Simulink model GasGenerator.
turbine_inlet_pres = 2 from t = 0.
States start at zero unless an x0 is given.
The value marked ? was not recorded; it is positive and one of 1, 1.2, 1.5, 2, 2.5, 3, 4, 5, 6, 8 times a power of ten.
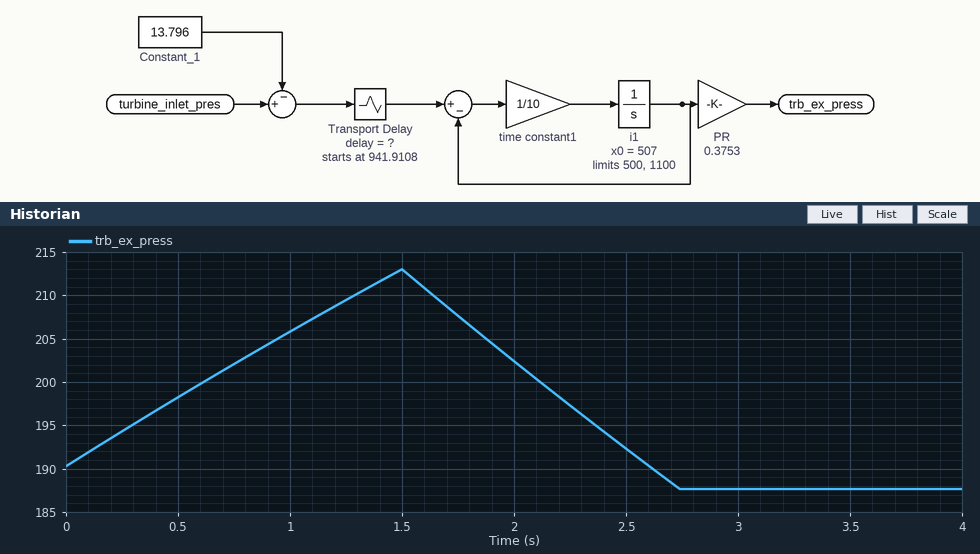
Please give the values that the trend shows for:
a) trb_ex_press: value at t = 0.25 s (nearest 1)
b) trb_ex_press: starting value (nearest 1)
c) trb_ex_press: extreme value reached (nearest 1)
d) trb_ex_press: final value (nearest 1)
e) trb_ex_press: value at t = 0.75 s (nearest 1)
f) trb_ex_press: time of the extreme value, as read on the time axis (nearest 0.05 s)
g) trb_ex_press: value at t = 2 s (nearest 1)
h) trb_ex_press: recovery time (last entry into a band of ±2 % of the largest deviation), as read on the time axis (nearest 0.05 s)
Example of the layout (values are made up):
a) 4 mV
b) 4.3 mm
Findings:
a) 194
b) 190
c) 213
d) 188
e) 202
f) 1.50 s
g) 202
h) 2.70 s
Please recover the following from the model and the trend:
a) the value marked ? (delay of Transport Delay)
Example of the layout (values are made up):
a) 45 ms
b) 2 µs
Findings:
a) 1.5
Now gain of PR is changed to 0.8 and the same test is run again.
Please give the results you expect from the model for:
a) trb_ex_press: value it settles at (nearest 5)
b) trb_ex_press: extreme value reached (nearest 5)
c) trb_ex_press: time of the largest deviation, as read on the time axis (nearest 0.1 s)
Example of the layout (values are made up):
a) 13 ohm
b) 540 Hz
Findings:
a) 400
b) 455
c) 1.5 s
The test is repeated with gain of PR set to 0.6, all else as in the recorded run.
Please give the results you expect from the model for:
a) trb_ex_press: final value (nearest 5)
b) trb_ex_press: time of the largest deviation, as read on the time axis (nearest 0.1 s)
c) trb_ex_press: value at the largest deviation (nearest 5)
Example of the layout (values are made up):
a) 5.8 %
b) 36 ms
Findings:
a) 300
b) 1.5 s
c) 340
